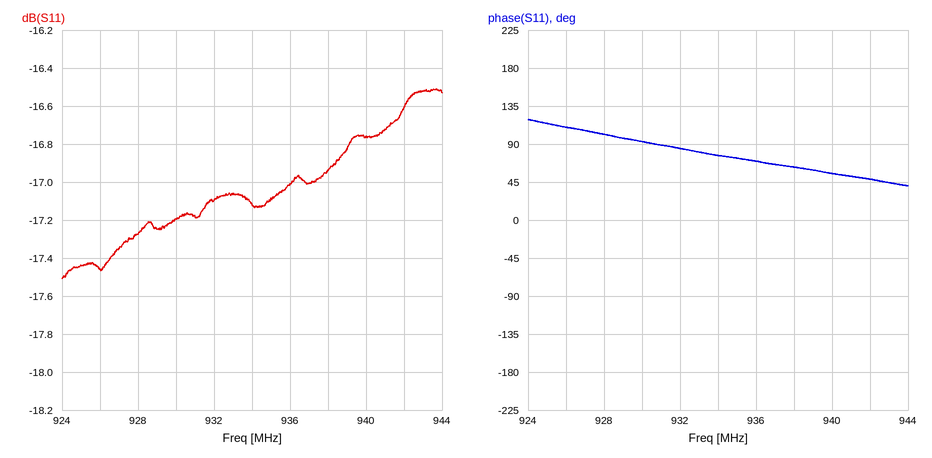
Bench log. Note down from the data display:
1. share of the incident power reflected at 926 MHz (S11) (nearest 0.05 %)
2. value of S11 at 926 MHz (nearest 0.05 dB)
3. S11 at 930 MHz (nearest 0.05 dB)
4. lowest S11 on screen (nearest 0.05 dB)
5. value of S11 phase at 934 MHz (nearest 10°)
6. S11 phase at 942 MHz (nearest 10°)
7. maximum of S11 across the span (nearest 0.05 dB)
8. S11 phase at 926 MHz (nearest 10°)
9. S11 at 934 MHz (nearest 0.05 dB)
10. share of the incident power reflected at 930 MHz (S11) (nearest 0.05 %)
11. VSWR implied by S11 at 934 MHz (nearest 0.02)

1.80 %
-17.45 dB
-17.20 dB
-17.50 dB
80°
50°
-16.50 dB
110°
-17.10 dB
1.90 %
1.32
